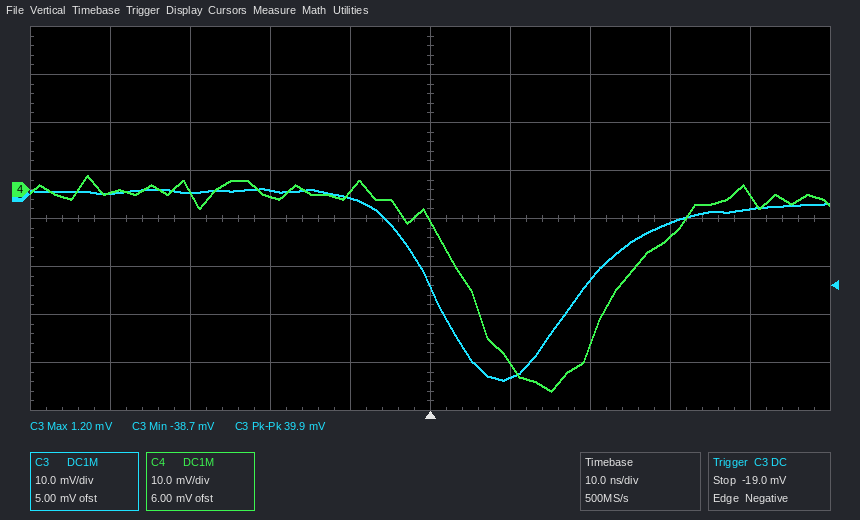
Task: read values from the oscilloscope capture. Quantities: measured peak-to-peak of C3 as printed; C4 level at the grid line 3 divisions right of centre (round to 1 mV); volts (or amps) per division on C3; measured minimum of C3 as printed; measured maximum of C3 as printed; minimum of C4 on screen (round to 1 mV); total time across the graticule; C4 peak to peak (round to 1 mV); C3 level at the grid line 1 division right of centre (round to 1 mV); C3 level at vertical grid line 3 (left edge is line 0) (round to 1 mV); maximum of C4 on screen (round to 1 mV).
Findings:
39.9 mV
-10 mV
10 mV
-38.7 mV
1.20 mV
-42 mV
100 ns
45 mV
-38 mV
1 mV
3 mV
